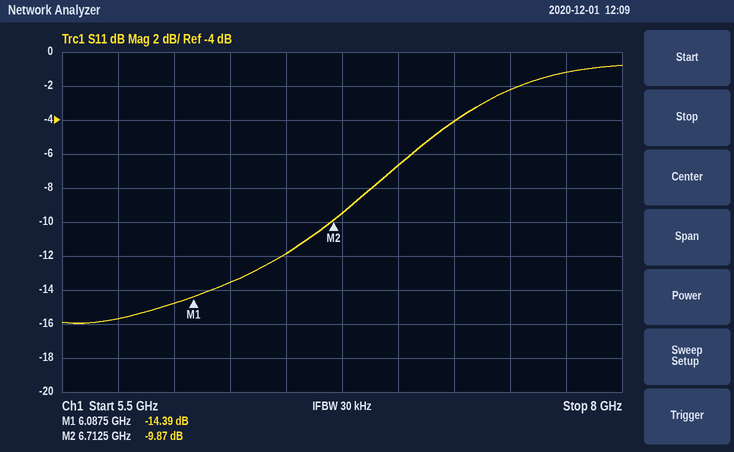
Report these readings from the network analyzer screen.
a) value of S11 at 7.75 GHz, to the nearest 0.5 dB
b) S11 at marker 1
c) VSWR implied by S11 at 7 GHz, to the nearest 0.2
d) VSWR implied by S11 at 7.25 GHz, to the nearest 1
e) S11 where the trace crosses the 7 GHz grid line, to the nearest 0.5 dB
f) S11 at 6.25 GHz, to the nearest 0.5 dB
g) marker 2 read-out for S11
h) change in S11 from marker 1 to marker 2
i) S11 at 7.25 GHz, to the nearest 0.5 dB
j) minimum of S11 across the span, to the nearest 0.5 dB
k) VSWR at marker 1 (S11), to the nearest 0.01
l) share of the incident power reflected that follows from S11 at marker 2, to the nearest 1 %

-1.0 dB
-14.39 dB
2.8
4
-6.5 dB
-13.5 dB
-9.87 dB
4.52 dB
-4.0 dB
-16.0 dB
1.47
10 %
